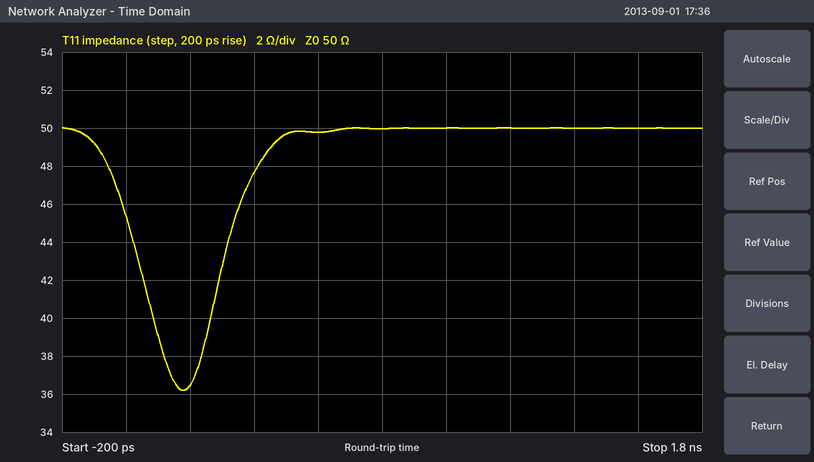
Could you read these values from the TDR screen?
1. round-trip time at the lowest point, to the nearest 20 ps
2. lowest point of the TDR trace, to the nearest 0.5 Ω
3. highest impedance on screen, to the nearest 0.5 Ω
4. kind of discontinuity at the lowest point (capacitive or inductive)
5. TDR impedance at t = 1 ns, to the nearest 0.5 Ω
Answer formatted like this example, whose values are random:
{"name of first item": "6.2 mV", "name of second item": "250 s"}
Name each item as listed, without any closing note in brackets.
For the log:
{"round-trip time at the lowest point, to the nearest 20 ps": "180 ps", "lowest point of the TDR trace, to the nearest 0.5 Ω": "36.0 Ω", "highest impedance on screen, to the nearest 0.5 Ω": "50.0 Ω", "kind of discontinuity at the lowest point": "capacitive", "TDR impedance at t = 1 ns, to the nearest 0.5 Ω": "50.0 Ω"}
